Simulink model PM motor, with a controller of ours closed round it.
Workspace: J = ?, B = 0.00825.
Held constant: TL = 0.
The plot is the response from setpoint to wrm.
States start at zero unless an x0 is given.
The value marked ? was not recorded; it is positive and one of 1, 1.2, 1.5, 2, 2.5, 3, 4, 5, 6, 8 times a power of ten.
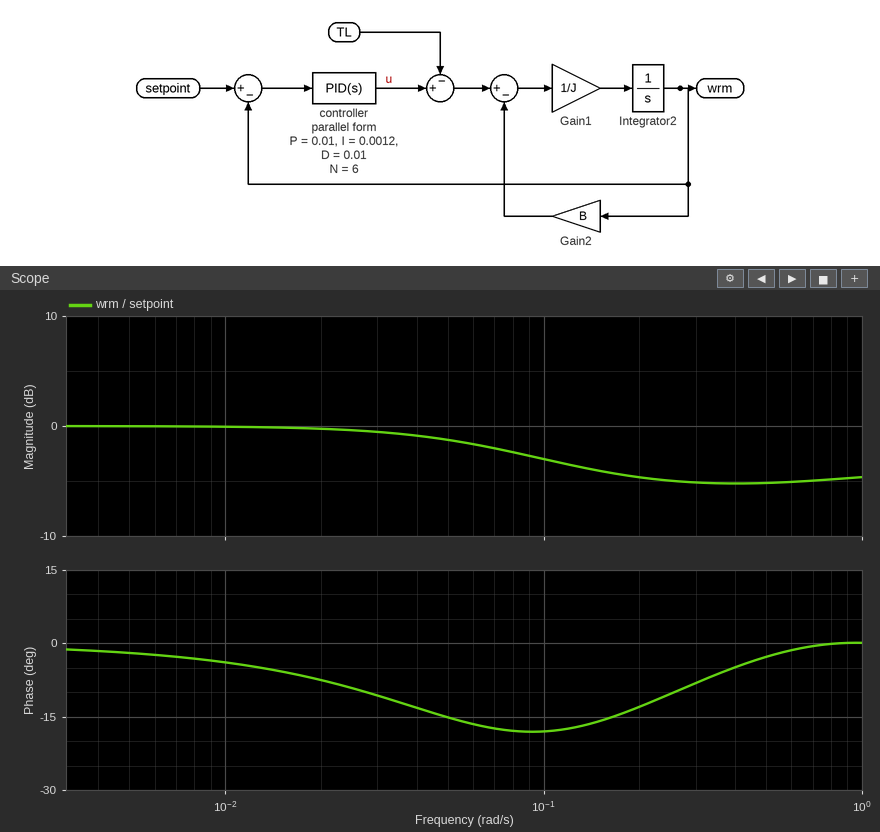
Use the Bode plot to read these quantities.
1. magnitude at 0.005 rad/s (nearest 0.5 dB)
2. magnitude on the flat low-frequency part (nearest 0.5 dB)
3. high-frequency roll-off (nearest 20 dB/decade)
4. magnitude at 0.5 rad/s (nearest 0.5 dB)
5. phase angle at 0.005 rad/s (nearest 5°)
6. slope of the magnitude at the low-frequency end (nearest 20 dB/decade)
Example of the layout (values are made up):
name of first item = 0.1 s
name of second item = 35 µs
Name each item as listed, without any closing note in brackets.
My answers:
magnitude at 0.005 rad/s = 0.0 dB
magnitude on the flat low-frequency part = 0.0 dB
high-frequency roll-off = 0 dB/decade
magnitude at 0.5 rad/s = -5.0 dB
phase angle at 0.005 rad/s = 0°
slope of the magnitude at the low-frequency end = 0 dB/decade
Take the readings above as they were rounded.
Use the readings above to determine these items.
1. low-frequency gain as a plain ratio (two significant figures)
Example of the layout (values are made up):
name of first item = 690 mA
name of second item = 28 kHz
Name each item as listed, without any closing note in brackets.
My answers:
low-frequency gain as a plain ratio = 1.0
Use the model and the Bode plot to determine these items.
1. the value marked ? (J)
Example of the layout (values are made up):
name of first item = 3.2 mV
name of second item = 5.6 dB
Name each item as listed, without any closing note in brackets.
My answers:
the value marked ? = 0.006
